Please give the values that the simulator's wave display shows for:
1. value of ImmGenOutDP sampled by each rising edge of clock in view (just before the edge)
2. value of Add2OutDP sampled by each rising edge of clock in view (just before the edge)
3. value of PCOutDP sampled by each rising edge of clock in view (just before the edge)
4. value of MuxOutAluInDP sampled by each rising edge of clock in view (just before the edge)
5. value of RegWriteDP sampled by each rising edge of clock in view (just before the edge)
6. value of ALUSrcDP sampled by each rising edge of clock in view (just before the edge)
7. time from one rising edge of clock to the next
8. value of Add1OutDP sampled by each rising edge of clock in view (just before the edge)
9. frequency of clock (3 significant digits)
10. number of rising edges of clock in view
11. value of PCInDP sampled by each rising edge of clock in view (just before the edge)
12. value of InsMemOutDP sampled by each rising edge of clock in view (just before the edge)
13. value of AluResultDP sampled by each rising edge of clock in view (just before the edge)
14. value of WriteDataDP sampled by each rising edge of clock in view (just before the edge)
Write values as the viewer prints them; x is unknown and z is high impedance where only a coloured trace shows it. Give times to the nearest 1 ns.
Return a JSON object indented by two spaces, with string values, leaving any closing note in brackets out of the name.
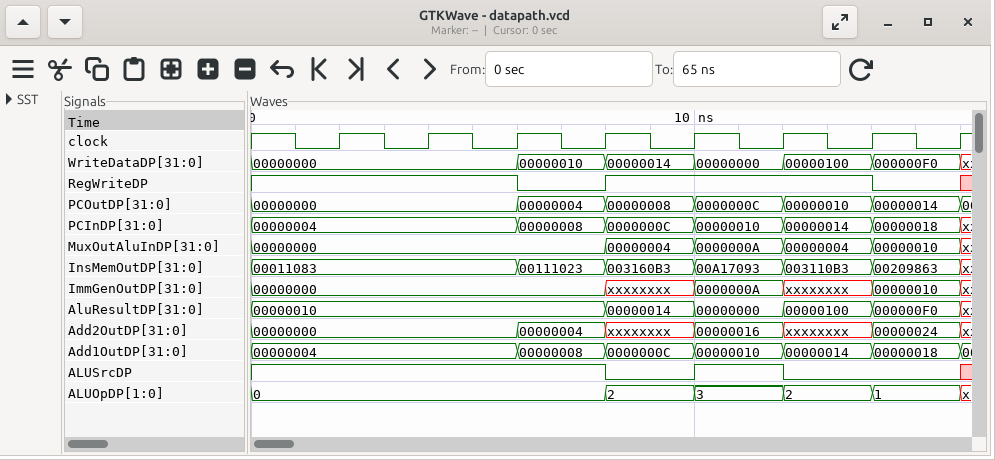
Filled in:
{
  "value of ImmGenOutDP sampled by each rising edge of clock in view": "00000000, 00000000, 00000000, 00000000, xxxxxxxx, 0000000A, xxxxxxxx, 00000010",
  "value of Add2OutDP sampled by each rising edge of clock in view": "00000000, 00000000, 00000000, 00000004, xxxxxxxx, 00000016, xxxxxxxx, 00000024",
  "value of PCOutDP sampled by each rising edge of clock in view": "00000000, 00000000, 00000000, 00000004, 00000008, 0000000C, 00000010, 00000014",
  "value of MuxOutAluInDP sampled by each rising edge of clock in view": "00000000, 00000000, 00000000, 00000000, 00000004, 0000000A, 00000004, 00000010",
  "value of RegWriteDP sampled by each rising edge of clock in view": "1 1 1 0 1 1 1 0",
  "value of ALUSrcDP sampled by each rising edge of clock in view": "1 1 1 1 0 1 0 0",
  "time from one rising edge of clock to the next": "2 ns",
  "value of Add1OutDP sampled by each rising edge of clock in view": "00000004, 00000004, 00000004, 00000008, 0000000C, 00000010, 00000014, 00000018",
  "frequency of clock": "500 MHz",
  "number of rising edges of clock in view": "8",
  "value of PCInDP sampled by each rising edge of clock in view": "00000004, 00000004, 00000004, 00000008, 0000000C, 00000010, 00000014, 00000018",
  "value of InsMemOutDP sampled by each rising edge of clock in view": "00011083, 00011083, 00011083, 00111023, 003160B3, 00A17093, 003110B3, 00209863",
  "value of AluResultDP sampled by each rising edge of clock in view": "00000010, 00000010, 00000010, 00000010, 00000014, 00000000, 00000100, 000000F0",
  "value of WriteDataDP sampled by each rising edge of clock in view": "00000000, 00000000, 00000000, 00000010, 00000014, 00000000, 00000100, 000000F0"
}
